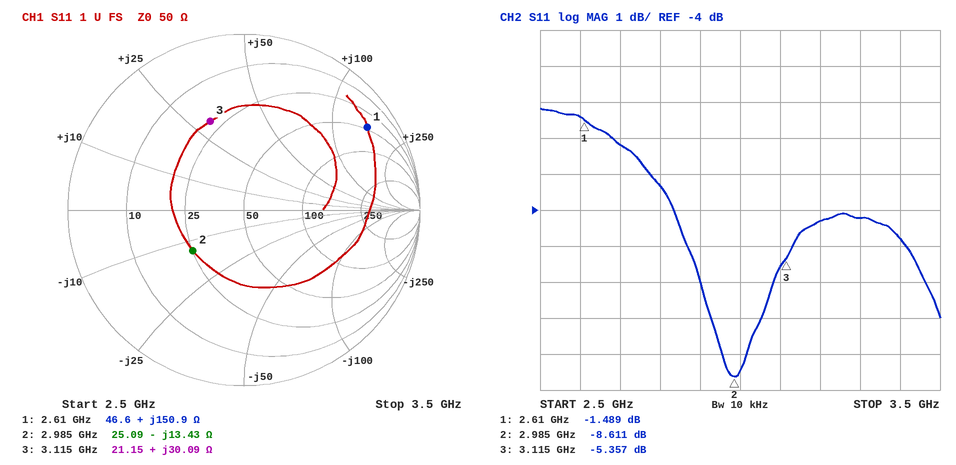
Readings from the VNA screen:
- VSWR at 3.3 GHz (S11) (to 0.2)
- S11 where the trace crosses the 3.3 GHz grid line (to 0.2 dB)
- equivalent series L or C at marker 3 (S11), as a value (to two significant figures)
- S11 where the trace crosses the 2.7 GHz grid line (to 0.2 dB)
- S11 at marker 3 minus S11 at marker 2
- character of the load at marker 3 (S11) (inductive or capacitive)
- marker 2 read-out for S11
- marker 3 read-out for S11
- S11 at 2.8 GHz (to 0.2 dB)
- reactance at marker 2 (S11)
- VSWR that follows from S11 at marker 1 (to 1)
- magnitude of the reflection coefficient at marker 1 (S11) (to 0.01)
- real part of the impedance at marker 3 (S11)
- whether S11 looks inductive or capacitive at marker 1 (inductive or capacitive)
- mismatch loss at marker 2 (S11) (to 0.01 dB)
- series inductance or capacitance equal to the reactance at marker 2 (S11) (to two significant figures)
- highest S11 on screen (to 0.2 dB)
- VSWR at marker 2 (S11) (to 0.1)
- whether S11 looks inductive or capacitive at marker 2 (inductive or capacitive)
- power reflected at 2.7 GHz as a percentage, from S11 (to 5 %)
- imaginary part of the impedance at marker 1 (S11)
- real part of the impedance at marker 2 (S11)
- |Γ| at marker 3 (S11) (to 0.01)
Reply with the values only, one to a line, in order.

4.2
-4.2 dB
1.5 nH
-2.2 dB
3.254 dB
inductive
-8.611 dB
-5.357 dB
-3.4 dB
-13.43 Ω
12
0.84
21.15 Ω
inductive
0.64 dB
4.0 pF
-1.2 dB
2.2
capacitive
60 %
+150.9 Ω
25.09 Ω
0.54
